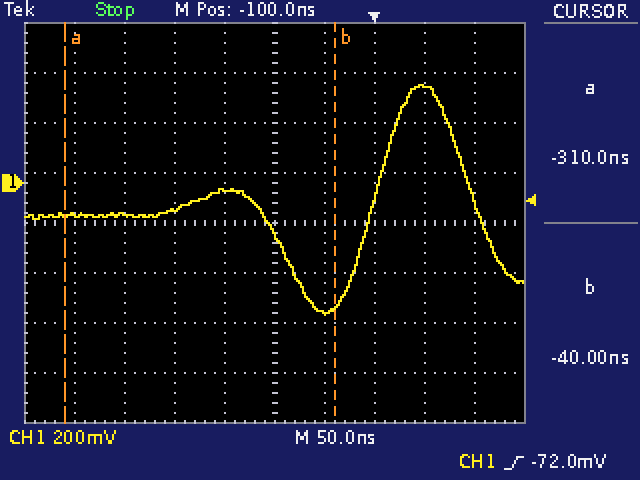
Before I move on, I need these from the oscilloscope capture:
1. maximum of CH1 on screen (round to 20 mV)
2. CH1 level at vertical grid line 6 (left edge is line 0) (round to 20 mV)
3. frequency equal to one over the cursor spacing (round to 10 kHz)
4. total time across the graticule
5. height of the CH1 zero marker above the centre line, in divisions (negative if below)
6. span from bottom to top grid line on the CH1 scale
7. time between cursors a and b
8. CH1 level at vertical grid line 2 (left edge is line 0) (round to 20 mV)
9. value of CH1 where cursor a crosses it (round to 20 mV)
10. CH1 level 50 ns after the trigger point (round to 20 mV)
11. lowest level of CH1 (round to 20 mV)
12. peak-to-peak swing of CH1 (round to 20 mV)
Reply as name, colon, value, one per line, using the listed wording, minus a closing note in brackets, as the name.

maximum of CH1 on screen: 400 mV
CH1 level at vertical grid line 6 (left edge is line 0): -520 mV
frequency equal to one over the cursor spacing: 3.70 MHz
total time across the graticule: 500 ns
height of the CH1 zero marker above the centre line, in divisions: +0.8 div
span from bottom to top grid line on the CH1 scale: 1.6 V
time between cursors a and b: 270 ns
CH1 level at vertical grid line 2 (left edge is line 0): -120 mV
value of CH1 where cursor a crosses it: -120 mV
CH1 level 50 ns after the trigger point: 380 mV
lowest level of CH1: -520 mV
peak-to-peak swing of CH1: 920 mV
